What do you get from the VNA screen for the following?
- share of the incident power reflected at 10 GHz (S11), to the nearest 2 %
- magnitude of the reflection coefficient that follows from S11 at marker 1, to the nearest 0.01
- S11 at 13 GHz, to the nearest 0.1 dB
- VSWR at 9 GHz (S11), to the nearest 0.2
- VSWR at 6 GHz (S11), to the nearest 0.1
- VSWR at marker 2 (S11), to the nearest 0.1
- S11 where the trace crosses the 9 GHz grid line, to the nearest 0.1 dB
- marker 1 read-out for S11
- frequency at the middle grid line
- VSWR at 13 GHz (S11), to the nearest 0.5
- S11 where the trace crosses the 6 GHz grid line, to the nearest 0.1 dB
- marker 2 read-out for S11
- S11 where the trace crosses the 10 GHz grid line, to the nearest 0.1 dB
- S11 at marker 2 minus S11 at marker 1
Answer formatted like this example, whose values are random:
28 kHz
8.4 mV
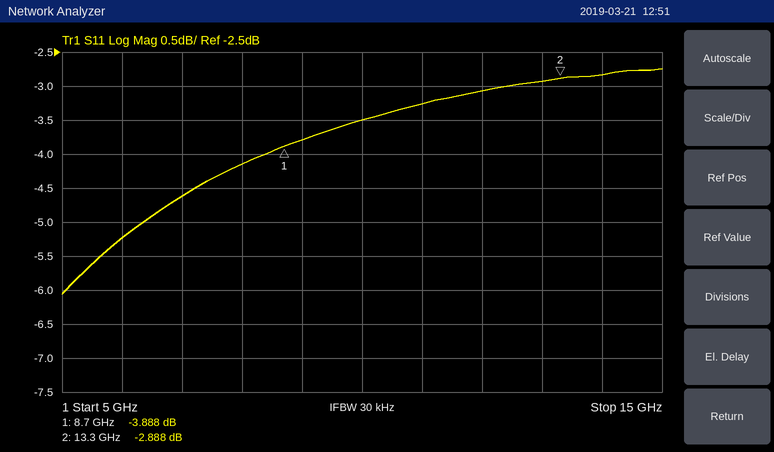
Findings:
44 %
0.64
-2.9 dB
4.6
3.4
6.1
-3.8 dB
-3.888 dB
10 GHz
6.0
-5.2 dB
-2.888 dB
-3.5 dB
1.000 dB
